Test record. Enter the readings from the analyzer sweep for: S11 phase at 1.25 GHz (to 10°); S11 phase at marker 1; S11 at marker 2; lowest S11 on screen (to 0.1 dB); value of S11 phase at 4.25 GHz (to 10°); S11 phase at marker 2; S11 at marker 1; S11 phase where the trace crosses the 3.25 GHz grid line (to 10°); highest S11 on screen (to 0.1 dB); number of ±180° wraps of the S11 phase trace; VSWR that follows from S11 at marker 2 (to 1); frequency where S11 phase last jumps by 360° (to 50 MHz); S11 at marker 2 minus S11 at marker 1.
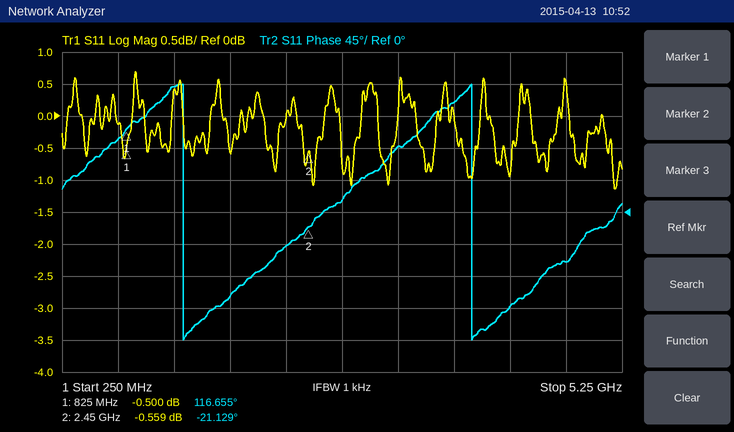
180°
116.655°
-0.559 dB
-1.1 dB
-130°
-21.129°
-0.500 dB
90°
0.7 dB
2
31
3.90 GHz
-0.059 dB
